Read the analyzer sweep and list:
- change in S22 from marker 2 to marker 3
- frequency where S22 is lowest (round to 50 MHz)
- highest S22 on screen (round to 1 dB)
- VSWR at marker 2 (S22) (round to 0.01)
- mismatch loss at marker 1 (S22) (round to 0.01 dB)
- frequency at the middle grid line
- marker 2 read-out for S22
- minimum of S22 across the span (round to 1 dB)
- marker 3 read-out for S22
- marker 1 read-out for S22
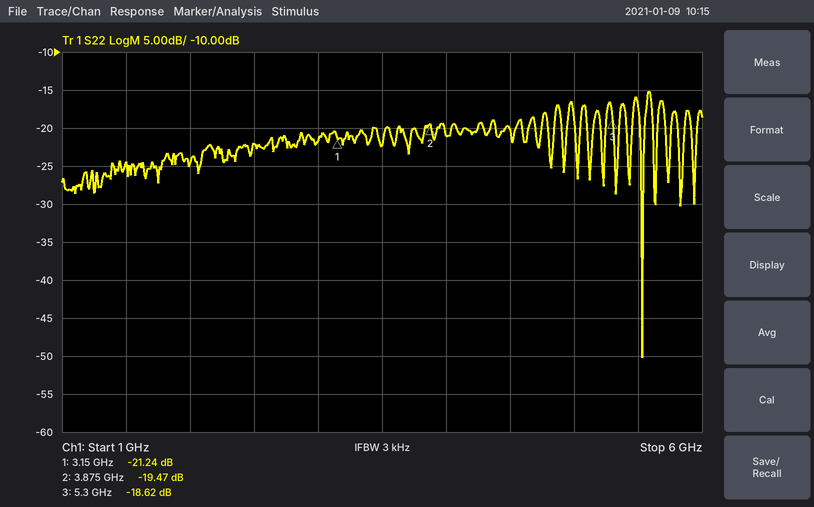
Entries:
0.85 dB
5.55 GHz
-15 dB
1.24
0.03 dB
3.5 GHz
-19.47 dB
-50 dB
-18.62 dB
-21.24 dB
